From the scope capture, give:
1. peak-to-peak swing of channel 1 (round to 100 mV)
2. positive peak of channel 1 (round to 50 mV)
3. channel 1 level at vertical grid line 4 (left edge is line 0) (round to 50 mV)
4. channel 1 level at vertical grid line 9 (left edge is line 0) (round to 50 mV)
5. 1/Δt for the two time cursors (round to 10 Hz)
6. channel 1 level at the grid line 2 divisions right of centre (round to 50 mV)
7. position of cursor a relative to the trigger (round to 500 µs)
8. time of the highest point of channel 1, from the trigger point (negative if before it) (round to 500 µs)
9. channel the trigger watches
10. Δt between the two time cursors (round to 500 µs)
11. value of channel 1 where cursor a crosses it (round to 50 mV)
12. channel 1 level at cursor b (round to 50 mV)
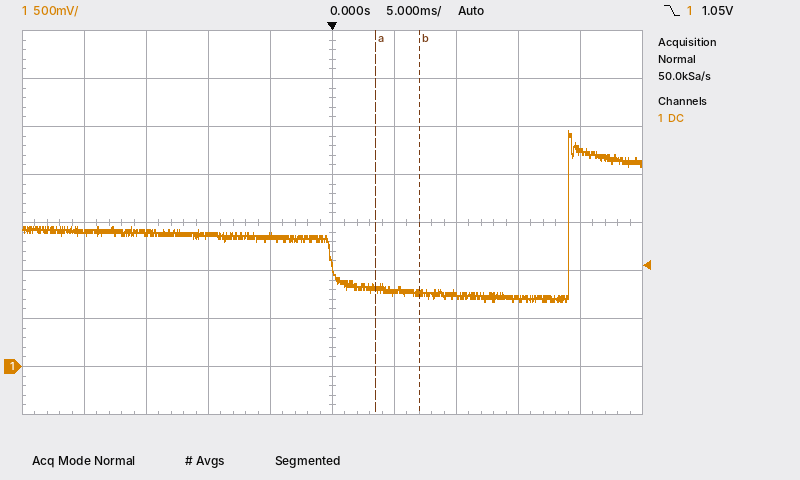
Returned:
1.80 V
2.45 V
1.35 V
2.25 V
290 Hz
750 mV
+3.5 ms
+19.0 ms
channel 1
3.5 ms
800 mV
750 mV
